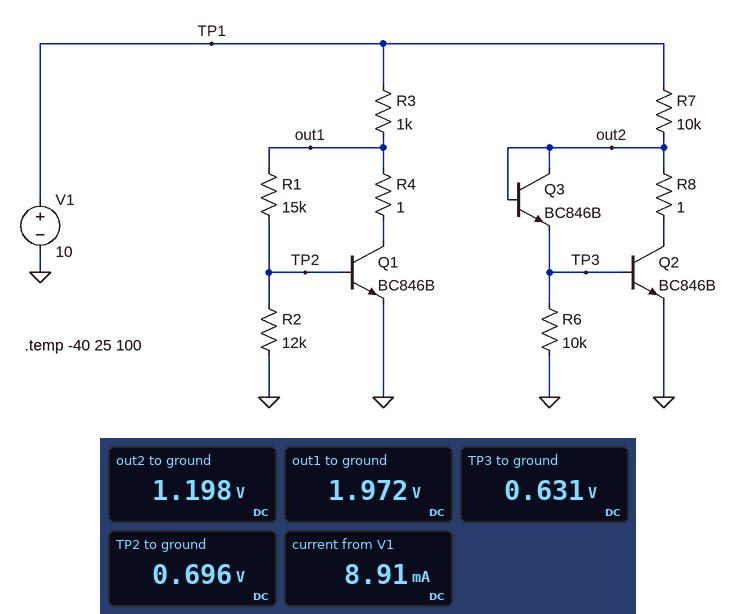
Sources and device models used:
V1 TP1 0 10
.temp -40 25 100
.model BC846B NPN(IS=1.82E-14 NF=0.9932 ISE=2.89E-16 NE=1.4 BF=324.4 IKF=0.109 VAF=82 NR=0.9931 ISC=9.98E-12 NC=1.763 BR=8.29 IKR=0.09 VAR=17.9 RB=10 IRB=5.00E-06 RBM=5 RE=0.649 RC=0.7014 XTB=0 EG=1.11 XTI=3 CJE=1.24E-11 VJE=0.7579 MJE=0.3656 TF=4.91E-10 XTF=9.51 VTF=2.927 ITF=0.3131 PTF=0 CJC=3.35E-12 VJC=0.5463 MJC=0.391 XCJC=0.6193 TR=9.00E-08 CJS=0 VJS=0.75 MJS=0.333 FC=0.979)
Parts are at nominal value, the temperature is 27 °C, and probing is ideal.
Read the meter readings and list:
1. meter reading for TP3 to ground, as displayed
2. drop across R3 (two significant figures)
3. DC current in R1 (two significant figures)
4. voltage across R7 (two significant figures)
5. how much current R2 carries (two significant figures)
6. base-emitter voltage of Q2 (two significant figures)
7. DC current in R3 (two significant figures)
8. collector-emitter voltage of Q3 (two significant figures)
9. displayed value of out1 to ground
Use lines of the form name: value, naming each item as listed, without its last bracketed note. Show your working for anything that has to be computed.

meter reading for TP3 to ground, as displayed: 0.631 V
drop across R3: 10 V - 1.972 V = 8.0 V
DC current in R1: (1.972 V - 696 mV) / 15 kΩ = 85 µA
voltage across R7: 10 V - 1.198 V = 8.8 V
how much current R2 carries: (696 mV) / 12 kΩ = 58 µA
base-emitter voltage of Q2: 631 mV = 630 mV
DC current in R3: (10 V - 1.972 V) / 1 kΩ = 8.0 mA
collector-emitter voltage of Q3: 1.198 V - 631 mV = 570 mV
displayed value of out1 to ground: 1.972 V
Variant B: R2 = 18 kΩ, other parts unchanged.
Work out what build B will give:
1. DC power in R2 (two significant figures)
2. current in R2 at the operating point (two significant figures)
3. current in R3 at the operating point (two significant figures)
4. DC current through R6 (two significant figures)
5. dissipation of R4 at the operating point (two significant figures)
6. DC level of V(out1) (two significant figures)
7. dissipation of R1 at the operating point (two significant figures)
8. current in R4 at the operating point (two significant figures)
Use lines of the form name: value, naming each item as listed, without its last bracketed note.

DC power in R2: 27 µW
current in R2 at the operating point: 39 µA
current in R3 at the operating point: 8.3 mA
DC current through R6: 63 µA
dissipation of R4 at the operating point: 68 µW
DC level of V(out1): 1.7 V
dissipation of R1 at the operating point: 67 µW
current in R4 at the operating point: 8.2 mA
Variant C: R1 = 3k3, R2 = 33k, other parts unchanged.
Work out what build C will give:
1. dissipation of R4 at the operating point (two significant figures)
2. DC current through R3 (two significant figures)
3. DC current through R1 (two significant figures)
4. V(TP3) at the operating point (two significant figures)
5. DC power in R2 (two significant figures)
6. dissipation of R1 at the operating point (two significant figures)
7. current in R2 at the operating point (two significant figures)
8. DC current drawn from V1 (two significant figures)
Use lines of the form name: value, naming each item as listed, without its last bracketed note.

dissipation of R4 at the operating point: 82 µW
DC current through R3: 9.1 mA
DC current through R1: 53 µA
V(TP3) at the operating point: 630 mV
DC power in R2: 15 µW
dissipation of R1 at the operating point: 9.2 µW
current in R2 at the operating point: 21 µA
DC current drawn from V1: 10 mA
